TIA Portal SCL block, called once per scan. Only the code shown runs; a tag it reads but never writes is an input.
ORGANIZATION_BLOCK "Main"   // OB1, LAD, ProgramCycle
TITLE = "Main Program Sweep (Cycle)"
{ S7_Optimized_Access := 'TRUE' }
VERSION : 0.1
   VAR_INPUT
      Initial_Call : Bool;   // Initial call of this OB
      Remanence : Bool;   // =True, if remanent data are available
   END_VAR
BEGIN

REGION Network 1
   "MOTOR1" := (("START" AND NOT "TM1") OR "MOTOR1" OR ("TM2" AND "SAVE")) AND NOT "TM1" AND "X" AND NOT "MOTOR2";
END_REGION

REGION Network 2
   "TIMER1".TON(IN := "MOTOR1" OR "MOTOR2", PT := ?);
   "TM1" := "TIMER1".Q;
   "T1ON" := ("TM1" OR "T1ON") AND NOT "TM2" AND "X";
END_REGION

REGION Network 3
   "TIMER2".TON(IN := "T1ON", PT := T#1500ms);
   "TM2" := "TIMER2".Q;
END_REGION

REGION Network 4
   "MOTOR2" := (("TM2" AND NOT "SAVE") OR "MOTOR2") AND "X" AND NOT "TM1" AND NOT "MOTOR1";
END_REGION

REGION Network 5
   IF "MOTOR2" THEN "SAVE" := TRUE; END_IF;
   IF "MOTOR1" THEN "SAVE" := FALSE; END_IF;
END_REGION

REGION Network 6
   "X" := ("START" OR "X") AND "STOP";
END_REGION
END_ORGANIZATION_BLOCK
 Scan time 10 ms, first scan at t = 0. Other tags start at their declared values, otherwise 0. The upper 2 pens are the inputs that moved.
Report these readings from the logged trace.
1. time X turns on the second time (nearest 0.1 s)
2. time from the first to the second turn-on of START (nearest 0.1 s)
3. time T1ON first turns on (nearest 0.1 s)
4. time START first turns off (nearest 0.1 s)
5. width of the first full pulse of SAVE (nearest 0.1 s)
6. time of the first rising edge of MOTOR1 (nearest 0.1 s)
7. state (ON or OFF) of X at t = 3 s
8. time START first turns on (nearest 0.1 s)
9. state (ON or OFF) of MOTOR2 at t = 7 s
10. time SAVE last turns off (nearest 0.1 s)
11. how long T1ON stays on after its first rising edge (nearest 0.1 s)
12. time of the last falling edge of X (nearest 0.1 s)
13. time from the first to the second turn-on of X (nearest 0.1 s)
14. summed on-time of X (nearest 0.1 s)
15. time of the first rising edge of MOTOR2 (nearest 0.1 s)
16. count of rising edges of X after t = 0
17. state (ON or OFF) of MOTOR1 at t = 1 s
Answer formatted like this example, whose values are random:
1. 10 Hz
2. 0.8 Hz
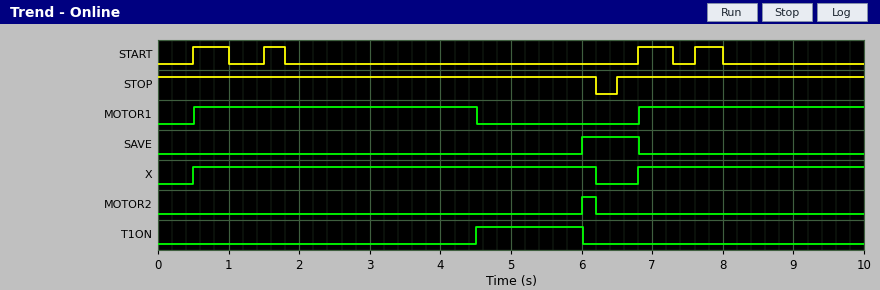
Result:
1. 6.8 s
2. 1.0 s
3. 4.5 s
4. 1.0 s
5. 0.8 s
6. 0.5 s
7. ON
8. 0.5 s
9. OFF
10. 6.8 s
11. 1.5 s
12. 6.2 s
13. 6.3 s
14. 8.9 s
15. 6.0 s
16. 2
17. ON
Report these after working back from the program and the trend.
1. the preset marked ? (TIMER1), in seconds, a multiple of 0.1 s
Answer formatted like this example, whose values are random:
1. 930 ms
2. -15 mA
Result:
1. 4.0 s
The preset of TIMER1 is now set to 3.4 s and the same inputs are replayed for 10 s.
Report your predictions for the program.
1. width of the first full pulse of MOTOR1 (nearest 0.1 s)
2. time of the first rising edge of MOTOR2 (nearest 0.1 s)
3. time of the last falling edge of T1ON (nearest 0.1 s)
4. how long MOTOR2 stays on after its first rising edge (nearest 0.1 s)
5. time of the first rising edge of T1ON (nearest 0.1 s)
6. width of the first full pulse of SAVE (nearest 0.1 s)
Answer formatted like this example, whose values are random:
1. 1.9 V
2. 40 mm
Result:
1. 3.4 s
2. 5.4 s
3. 5.4 s
4. 0.8 s
5. 3.9 s
6. 1.4 s
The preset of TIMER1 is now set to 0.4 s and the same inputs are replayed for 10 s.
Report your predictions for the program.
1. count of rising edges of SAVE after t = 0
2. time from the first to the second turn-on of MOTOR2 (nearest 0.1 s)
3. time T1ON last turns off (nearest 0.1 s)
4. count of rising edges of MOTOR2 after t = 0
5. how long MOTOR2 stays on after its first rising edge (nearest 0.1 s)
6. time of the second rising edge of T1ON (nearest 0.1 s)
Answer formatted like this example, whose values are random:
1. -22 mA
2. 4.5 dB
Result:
1. 2
2. 6.3 s
3. 8.7 s
4. 2
5. 0.4 s
6. 2.8 s
